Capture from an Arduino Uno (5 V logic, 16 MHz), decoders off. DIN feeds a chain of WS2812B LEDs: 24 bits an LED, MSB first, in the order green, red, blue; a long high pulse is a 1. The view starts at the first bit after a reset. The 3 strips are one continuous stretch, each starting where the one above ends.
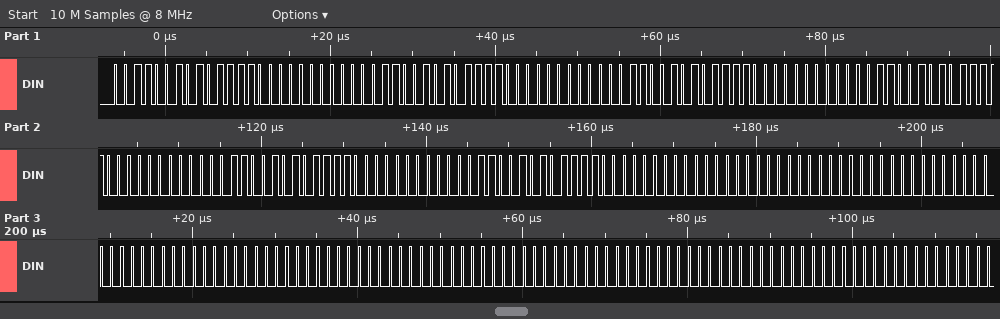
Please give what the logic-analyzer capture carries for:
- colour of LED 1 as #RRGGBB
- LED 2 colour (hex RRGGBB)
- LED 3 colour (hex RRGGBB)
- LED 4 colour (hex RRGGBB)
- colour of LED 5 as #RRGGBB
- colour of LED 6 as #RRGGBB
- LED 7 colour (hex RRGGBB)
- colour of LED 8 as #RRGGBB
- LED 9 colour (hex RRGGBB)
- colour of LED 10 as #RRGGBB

#BC3200
#BC3200
#BC3200
#BC3200
#BC3200
#BC3200
#000000
#000000
#000000
#000000
